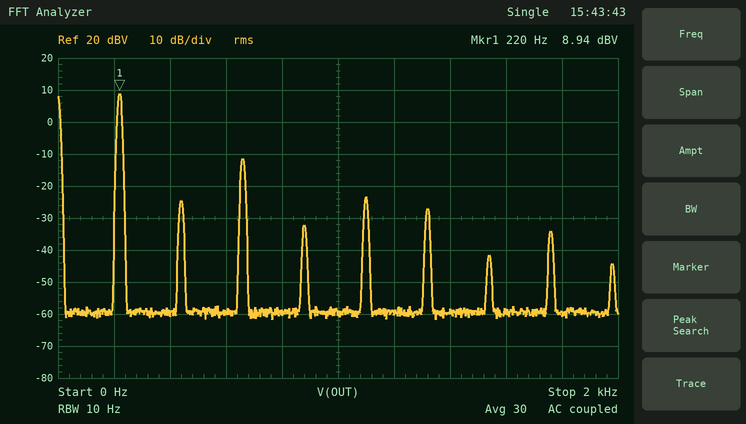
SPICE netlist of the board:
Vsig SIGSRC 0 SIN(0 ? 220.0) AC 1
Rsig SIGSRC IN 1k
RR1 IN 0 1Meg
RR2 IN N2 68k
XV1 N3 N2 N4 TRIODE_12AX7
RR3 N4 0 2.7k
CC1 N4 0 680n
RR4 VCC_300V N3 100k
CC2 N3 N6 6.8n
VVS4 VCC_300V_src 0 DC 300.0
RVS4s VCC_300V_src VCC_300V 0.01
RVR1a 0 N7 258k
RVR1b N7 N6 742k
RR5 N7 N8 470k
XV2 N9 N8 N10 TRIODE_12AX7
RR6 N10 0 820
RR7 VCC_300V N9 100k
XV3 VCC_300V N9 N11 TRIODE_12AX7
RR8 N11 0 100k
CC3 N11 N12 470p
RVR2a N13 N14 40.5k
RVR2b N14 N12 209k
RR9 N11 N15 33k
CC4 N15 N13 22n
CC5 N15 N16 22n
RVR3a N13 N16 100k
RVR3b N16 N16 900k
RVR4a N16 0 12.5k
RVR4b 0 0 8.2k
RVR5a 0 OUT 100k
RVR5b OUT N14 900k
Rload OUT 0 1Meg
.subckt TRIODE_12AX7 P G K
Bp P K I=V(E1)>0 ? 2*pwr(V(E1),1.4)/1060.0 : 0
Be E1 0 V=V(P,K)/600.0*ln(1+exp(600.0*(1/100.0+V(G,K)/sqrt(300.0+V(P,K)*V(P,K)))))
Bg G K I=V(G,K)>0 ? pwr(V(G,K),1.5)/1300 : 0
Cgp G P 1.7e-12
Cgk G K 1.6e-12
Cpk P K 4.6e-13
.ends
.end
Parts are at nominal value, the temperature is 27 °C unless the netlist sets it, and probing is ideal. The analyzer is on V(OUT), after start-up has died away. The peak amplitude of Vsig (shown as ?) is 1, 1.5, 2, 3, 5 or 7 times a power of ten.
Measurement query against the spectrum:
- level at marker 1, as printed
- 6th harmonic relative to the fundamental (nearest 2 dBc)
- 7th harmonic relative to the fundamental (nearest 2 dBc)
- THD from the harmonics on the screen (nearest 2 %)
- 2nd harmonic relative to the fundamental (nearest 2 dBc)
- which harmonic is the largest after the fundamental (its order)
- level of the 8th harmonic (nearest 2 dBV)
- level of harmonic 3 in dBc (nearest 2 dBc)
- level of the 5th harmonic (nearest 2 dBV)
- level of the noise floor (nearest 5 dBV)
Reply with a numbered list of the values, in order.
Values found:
1. 8.94 dBV
2. -36 dBc
3. -50 dBc
4. 10 %
5. -34 dBc
6. 3
7. -34 dBV
8. -20 dBc
9. -24 dBV
10. -60 dBV
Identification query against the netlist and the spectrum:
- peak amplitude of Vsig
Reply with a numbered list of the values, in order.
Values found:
1. 300 mV
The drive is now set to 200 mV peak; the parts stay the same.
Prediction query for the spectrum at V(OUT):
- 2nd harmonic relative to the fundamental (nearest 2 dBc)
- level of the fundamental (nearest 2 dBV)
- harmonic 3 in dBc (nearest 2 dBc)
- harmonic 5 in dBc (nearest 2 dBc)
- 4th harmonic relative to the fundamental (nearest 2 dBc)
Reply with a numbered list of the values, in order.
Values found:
1. -28 dBc
2. 8 dBV
3. -26 dBc
4. -58 dBc
5. -34 dBc
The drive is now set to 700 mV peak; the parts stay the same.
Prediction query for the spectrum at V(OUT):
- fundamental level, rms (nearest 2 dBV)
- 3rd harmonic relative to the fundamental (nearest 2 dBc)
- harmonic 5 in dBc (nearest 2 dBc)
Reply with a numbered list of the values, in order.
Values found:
1. 10 dBV
2. -16 dBc
3. -22 dBc
